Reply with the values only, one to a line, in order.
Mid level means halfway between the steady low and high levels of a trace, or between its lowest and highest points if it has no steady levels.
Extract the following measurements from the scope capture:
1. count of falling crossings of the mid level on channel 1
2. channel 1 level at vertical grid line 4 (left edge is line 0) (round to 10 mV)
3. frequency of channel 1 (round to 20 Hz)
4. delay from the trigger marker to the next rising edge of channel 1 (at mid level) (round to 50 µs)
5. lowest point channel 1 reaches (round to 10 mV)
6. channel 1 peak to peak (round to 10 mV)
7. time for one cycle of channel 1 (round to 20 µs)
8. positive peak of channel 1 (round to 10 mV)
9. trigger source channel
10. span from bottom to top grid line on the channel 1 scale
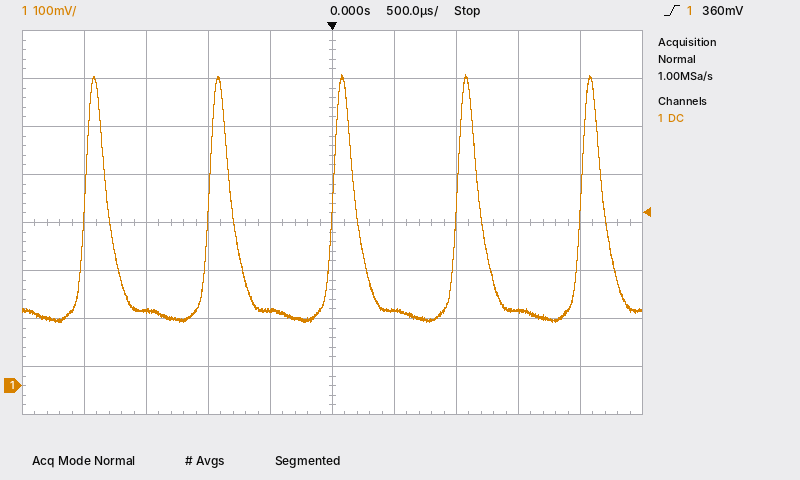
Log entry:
5
160 mV
1.00 kHz
1.00 ms
130 mV
520 mV
1.00 ms
650 mV
channel 1
800 mV
